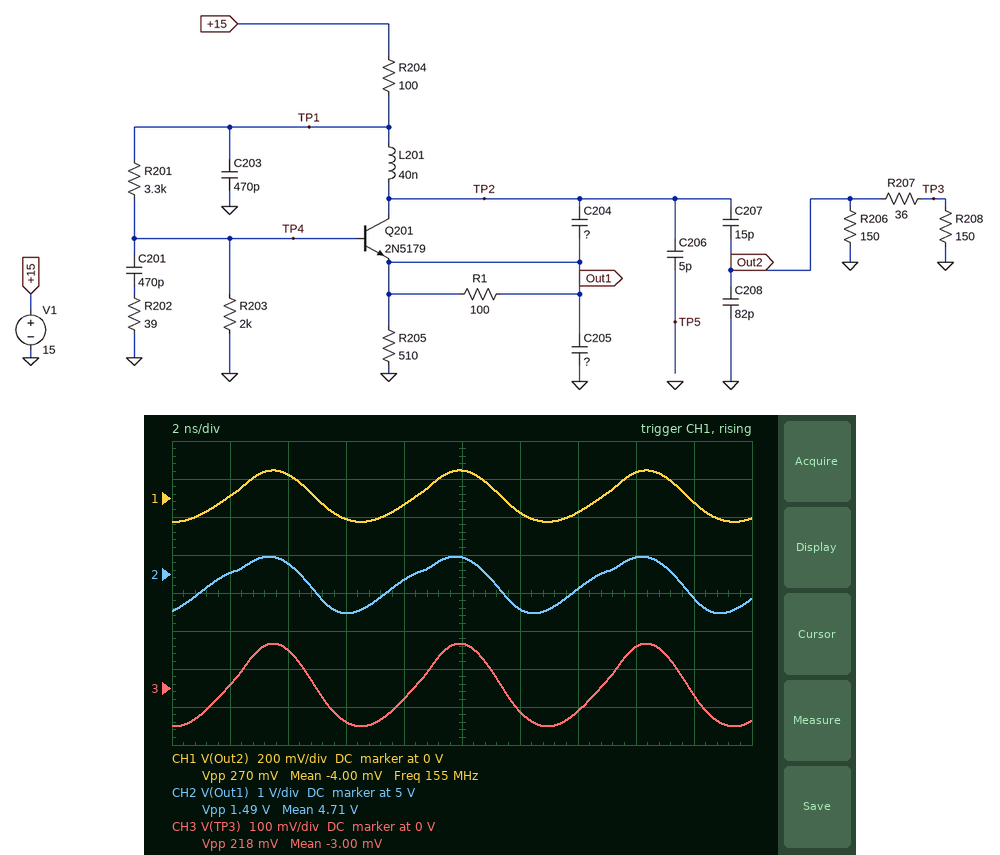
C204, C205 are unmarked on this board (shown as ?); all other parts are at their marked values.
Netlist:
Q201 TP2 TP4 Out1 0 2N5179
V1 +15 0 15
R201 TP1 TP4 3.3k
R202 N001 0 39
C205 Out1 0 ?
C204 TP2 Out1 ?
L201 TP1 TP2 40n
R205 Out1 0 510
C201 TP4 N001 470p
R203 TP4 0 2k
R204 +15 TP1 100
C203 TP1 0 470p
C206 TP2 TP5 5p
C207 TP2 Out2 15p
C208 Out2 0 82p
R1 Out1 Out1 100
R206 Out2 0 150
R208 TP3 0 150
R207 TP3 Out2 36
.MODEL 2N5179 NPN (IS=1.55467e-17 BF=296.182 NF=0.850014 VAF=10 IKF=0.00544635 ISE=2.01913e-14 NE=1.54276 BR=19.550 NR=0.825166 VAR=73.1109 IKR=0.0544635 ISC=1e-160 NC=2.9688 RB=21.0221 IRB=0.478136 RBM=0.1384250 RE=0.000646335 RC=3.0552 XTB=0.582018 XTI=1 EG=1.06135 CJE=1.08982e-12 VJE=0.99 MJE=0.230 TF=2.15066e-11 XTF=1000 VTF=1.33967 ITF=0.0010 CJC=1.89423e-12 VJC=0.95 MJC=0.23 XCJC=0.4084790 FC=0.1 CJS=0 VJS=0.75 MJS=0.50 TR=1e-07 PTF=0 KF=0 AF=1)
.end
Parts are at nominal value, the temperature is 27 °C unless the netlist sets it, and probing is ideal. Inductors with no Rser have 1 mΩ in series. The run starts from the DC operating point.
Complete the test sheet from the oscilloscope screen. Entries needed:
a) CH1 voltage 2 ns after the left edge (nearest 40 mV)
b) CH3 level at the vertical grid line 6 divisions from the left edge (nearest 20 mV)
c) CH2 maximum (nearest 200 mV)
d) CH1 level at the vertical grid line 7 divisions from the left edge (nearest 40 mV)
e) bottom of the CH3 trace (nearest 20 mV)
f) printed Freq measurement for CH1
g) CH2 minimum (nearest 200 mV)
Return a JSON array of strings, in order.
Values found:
["0 V", "-60 mV", "5.4 V", "-80 mV", "-100 mV", "155 MHz", "4.0 V"]
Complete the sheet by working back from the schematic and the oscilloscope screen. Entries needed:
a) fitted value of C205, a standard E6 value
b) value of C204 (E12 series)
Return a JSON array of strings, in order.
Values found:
["10 pF", "39 pF"]
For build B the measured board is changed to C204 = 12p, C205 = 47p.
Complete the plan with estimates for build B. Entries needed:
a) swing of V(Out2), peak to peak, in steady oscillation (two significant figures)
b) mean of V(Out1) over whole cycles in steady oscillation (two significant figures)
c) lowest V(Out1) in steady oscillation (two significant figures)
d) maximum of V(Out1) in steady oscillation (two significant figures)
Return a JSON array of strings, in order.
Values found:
["1.1 V", "4.7 V", "3.8 V", "5.6 V"]
